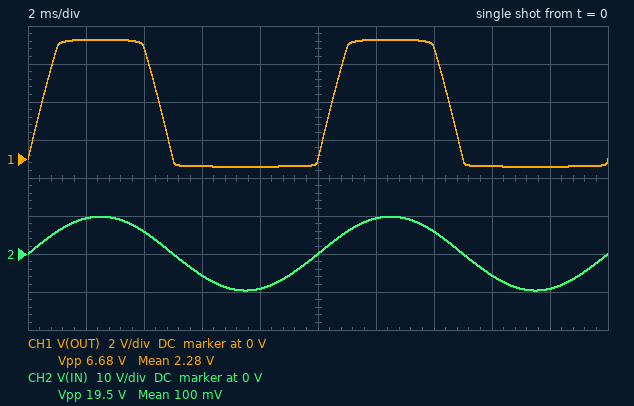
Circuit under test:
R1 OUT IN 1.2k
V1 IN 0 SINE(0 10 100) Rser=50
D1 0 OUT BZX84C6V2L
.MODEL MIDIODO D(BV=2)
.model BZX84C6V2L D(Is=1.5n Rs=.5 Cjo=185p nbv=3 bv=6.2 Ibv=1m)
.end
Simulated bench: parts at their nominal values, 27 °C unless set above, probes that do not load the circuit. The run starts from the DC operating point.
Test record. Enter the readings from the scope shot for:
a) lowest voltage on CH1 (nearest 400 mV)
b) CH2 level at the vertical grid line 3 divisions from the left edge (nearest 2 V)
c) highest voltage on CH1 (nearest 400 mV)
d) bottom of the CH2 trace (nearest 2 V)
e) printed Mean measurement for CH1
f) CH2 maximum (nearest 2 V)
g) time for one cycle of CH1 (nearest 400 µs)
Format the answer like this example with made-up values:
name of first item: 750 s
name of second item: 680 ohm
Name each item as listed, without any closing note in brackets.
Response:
lowest voltage on CH1: -400 mV
CH2 level at the vertical grid line 3 divisions from the left edge: -6 V
highest voltage on CH1: 6.4 V
bottom of the CH2 trace: -10 V
printed Mean measurement for CH1: 2.28 V
CH2 maximum: 10 V
time for one cycle of CH1: 10.0 ms
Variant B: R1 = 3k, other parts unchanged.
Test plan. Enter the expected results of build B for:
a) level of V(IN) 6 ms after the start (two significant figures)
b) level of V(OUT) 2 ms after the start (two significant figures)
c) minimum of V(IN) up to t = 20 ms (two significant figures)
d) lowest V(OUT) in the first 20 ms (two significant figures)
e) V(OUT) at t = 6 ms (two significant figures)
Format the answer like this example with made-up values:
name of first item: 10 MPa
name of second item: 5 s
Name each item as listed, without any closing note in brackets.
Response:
level of V(IN) 6 ms after the start: -5.8 V
level of V(OUT) 2 ms after the start: 6.2 V
minimum of V(IN) up to t = 20 ms: -9.8 V
lowest V(OUT) in the first 20 ms: -380 mV
V(OUT) at t = 6 ms: -360 mV
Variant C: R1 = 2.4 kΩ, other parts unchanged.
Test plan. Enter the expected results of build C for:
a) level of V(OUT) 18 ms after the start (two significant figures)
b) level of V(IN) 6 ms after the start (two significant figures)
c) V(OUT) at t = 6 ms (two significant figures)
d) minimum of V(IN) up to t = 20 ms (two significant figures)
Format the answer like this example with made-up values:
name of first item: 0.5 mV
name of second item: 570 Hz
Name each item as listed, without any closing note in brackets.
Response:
level of V(OUT) 18 ms after the start: -380 mV
level of V(IN) 6 ms after the start: -5.8 V
V(OUT) at t = 6 ms: -370 mV
minimum of V(IN) up to t = 20 ms: -9.8 V
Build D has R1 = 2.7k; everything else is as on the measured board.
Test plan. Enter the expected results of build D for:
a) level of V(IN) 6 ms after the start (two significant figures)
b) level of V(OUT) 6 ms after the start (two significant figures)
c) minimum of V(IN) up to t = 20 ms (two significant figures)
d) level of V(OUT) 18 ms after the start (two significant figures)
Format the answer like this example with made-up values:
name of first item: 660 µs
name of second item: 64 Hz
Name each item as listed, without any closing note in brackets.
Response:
level of V(IN) 6 ms after the start: -5.8 V
level of V(OUT) 6 ms after the start: -370 mV
minimum of V(IN) up to t = 20 ms: -9.8 V
level of V(OUT) 18 ms after the start: -380 mV
